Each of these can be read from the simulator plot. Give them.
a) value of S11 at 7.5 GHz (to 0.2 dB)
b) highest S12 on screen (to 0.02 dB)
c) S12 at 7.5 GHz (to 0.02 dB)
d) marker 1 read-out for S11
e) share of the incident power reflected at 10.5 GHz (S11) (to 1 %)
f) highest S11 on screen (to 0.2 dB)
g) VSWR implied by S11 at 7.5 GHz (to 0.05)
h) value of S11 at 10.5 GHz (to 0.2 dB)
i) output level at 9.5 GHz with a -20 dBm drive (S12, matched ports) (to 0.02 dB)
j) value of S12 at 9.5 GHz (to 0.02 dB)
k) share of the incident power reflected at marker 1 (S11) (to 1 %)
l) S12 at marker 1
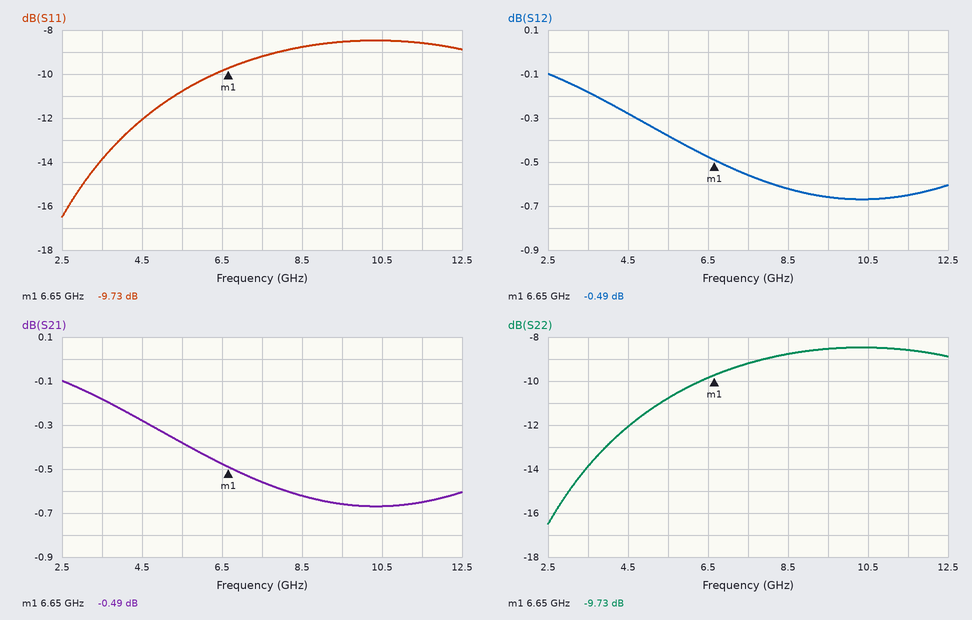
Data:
-9.2 dB
-0.10 dB
-0.56 dB
-9.73 dB
14 %
-8.4 dB
2.05
-8.4 dB
-20.66 dBm
-0.66 dB
11 %
-0.49 dB
